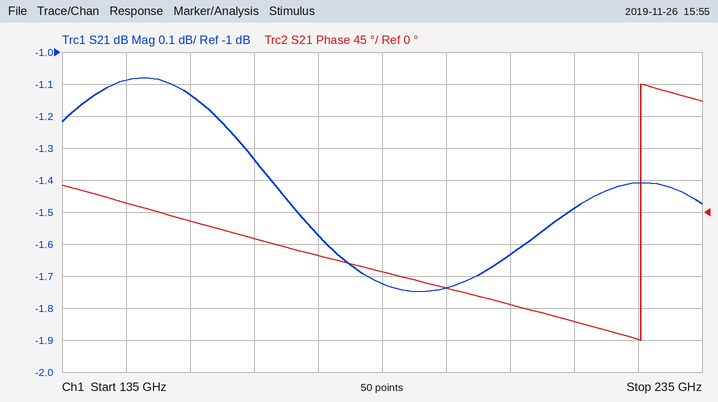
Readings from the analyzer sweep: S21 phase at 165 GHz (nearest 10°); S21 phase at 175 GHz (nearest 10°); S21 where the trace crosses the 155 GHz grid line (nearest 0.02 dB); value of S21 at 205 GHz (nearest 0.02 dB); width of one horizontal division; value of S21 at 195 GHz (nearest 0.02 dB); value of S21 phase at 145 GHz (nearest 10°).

-40°
-60°
-1.14 dB
-1.64 dB
10 GHz
-1.74 dB
10°
